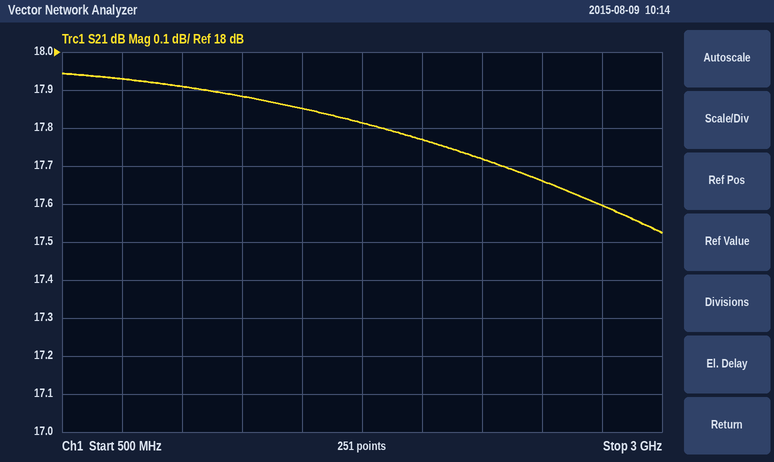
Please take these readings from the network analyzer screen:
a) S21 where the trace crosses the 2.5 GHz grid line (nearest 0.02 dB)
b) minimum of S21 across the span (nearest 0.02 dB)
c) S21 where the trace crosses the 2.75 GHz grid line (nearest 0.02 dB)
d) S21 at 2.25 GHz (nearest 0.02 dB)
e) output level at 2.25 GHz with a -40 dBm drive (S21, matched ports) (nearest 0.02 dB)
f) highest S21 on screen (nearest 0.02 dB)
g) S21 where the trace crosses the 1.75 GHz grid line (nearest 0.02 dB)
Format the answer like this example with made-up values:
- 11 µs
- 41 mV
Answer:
- 17.66 dB
- 17.52 dB
- 17.60 dB
- 17.72 dB
- -22.28 dBm
- 17.94 dB
- 17.82 dB
